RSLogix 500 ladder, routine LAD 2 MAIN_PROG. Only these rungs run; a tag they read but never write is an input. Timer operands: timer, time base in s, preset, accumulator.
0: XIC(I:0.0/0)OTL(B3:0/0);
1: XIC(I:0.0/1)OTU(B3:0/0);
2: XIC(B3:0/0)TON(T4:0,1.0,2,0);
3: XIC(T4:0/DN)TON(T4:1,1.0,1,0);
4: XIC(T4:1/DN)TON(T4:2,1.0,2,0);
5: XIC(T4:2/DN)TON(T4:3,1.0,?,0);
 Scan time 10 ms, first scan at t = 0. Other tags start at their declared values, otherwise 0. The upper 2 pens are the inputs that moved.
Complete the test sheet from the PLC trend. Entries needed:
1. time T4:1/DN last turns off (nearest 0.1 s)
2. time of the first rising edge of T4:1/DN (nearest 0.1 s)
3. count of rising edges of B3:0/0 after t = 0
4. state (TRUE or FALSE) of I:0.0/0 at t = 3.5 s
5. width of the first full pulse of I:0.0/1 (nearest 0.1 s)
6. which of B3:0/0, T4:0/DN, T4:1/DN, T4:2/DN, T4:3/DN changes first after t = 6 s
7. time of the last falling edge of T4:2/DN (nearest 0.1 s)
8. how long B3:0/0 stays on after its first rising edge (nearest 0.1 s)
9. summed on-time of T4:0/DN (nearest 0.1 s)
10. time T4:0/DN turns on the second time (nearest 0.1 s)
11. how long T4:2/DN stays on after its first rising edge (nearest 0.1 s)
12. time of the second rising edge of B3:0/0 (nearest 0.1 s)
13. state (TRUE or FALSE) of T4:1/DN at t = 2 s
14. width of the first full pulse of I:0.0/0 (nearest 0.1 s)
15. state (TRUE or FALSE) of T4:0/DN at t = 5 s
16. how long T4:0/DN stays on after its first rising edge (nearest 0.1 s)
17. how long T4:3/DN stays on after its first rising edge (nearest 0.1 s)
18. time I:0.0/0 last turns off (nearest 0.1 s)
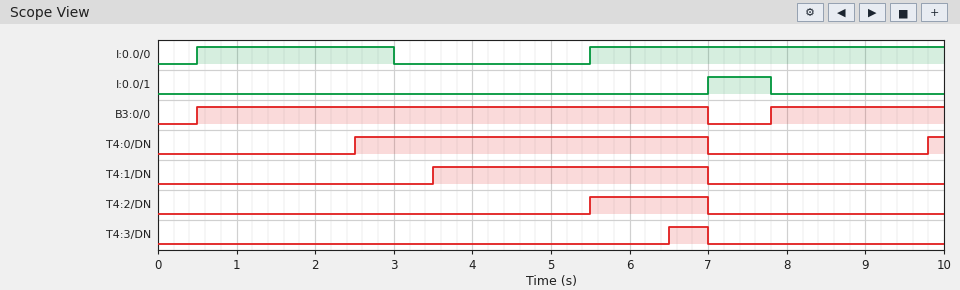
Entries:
7.0 s
3.5 s
2
FALSE
0.8 s
T4:3/DN
7.0 s
6.5 s
4.7 s
9.8 s
1.5 s
7.8 s
FALSE
2.5 s
TRUE
4.5 s
0.5 s
3.0 s
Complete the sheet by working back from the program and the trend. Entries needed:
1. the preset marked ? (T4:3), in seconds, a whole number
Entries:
1 s
